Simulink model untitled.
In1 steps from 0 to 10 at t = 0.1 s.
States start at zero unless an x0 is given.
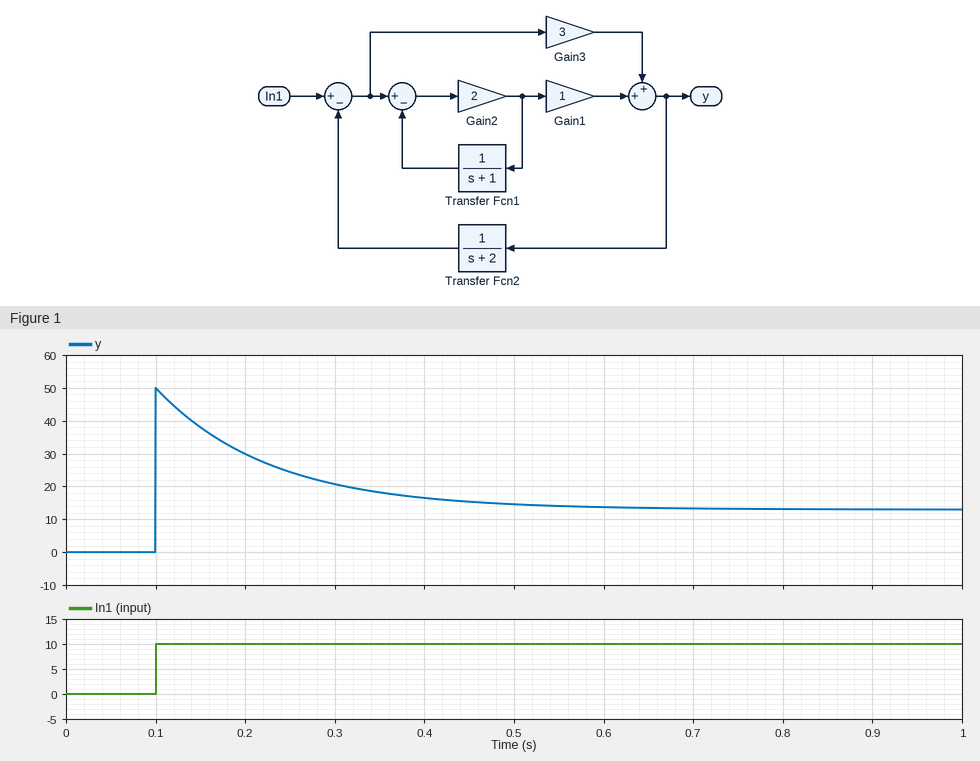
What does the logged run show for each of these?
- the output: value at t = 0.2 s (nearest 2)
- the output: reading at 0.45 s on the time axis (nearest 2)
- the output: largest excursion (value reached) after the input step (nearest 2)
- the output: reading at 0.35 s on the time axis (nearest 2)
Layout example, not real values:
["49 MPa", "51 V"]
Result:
["30", "16", "50", "18"]
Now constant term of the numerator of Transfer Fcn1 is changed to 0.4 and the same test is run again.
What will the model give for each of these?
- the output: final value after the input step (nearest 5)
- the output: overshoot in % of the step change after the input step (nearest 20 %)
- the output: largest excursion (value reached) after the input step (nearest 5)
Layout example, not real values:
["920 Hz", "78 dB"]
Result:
["15", "280 %", "50"]
